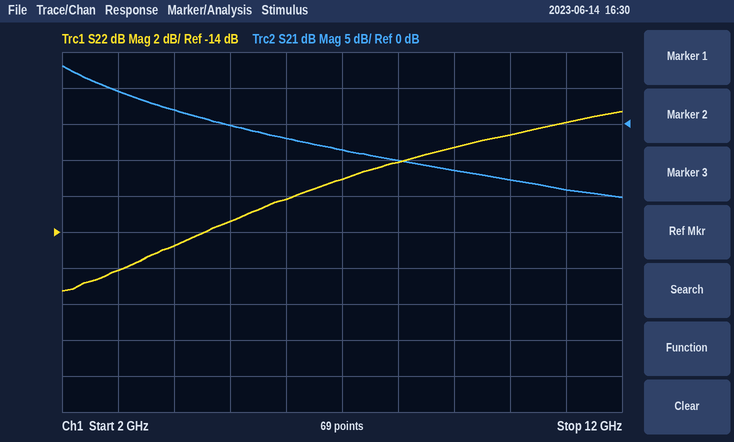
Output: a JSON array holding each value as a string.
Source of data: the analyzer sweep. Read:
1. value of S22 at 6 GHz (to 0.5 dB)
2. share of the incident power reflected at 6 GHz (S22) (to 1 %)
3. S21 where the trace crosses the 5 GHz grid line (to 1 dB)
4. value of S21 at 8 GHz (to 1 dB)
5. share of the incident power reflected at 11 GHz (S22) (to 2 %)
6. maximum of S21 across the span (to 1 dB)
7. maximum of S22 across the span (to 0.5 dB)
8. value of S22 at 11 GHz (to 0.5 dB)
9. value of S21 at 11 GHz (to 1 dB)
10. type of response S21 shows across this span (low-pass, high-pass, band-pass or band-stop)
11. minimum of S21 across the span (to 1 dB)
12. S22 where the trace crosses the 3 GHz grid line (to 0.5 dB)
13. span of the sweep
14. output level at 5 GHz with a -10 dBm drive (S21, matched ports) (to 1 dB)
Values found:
["-12.0 dB", "6 %", "0 dB", "-5 dB", "16 %", "8 dB", "-7.5 dB", "-8.0 dB", "-9 dB", "low-pass", "-10 dB", "-16.0 dB", "10 GHz", "-10 dBm"]
